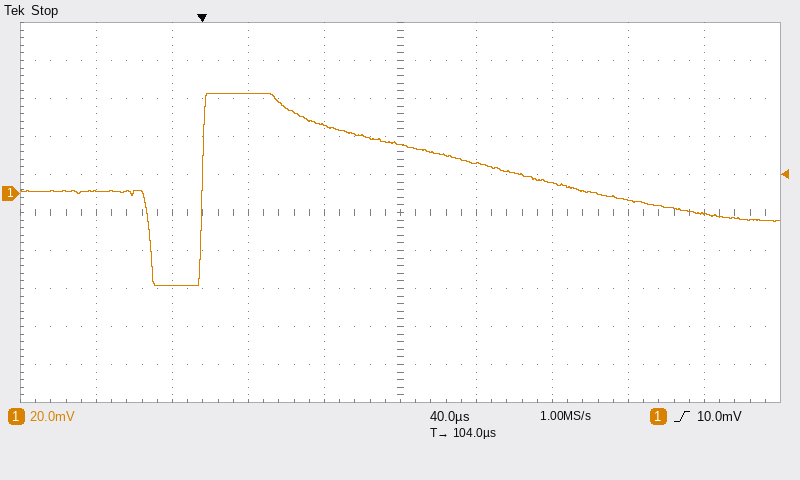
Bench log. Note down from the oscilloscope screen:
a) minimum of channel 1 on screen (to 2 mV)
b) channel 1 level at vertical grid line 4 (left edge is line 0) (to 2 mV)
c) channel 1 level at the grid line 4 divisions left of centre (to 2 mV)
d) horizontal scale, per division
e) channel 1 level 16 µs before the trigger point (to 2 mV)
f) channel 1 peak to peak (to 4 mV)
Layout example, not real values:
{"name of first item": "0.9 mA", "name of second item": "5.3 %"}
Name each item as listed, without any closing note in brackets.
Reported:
{"minimum of channel 1 on screen": "-48 mV", "channel 1 level at vertical grid line 4 (left edge is line 0)": "36 mV", "channel 1 level at the grid line 4 divisions left of centre": "2 mV", "horizontal scale, per division": "40 µs", "channel 1 level 16 µs before the trigger point": "-48 mV", "channel 1 peak to peak": "100 mV"}
